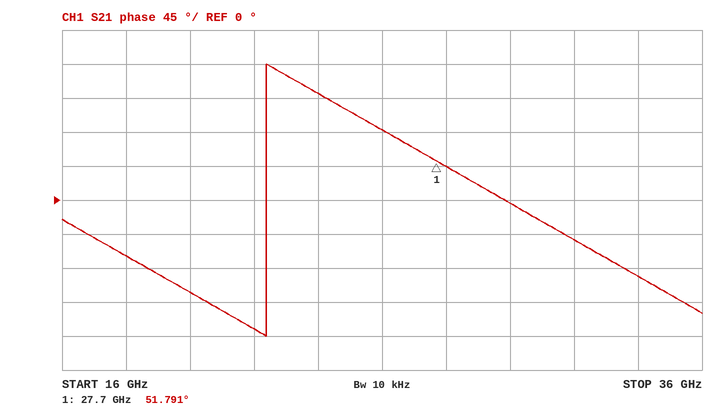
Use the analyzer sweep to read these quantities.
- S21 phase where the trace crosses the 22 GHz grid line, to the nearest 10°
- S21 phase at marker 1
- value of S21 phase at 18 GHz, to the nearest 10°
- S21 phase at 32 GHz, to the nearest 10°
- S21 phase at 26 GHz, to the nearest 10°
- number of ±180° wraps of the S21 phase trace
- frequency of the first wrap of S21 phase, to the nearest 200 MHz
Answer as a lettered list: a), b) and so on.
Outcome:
a) -170°
b) 51.791°
c) -70°
d) -50°
e) 90°
f) 1
g) 22.4 GHz
